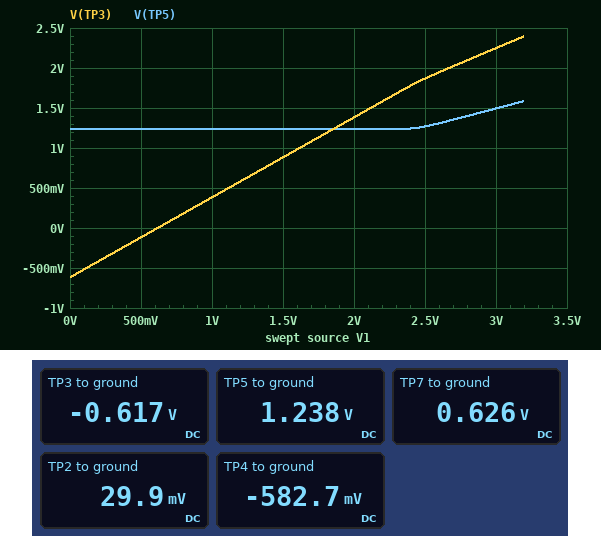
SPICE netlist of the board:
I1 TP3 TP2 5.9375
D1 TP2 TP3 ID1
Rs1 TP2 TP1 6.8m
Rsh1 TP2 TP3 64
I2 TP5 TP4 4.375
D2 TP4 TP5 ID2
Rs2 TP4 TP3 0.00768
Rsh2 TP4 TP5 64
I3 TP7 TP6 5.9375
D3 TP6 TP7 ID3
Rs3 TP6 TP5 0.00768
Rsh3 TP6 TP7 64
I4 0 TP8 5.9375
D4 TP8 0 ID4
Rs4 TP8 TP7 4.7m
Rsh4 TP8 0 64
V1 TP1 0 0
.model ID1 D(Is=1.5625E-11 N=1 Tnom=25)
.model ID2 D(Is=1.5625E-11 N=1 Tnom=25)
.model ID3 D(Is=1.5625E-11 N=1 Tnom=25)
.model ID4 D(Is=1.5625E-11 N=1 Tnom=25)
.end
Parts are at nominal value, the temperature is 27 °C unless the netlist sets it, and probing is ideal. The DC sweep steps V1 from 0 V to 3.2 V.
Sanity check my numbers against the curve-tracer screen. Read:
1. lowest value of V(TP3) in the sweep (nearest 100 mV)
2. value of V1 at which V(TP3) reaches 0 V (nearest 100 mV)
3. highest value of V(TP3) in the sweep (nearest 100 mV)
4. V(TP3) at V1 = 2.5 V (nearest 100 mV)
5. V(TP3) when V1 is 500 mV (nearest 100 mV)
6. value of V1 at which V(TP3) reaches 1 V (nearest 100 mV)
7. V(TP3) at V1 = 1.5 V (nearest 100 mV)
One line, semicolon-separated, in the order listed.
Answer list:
-600 mV; 600 mV; 2.4 V; 1.9 V; -100 mV; 1.6 V; 900 mV
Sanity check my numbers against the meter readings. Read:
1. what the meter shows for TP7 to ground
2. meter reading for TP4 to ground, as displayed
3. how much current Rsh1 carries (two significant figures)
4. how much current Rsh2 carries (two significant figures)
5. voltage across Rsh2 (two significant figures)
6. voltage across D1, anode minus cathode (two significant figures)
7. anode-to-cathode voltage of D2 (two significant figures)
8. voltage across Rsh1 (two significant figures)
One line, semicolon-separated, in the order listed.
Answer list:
0.626 V; -582.7 mV; 10 mA; 28 mA; 1.8 V; 650 mV; -1.8 V; 650 mV
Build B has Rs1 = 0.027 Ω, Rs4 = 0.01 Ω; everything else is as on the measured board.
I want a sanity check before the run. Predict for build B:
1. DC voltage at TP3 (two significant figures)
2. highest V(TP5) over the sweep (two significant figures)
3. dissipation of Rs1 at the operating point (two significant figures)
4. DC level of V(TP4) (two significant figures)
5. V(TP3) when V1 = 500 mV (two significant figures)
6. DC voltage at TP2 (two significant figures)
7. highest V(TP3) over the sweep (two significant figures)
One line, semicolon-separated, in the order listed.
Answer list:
-530 mV; 1.5 V; 520 mW; -490 mV; -28 mV; 120 mV; 2.3 V
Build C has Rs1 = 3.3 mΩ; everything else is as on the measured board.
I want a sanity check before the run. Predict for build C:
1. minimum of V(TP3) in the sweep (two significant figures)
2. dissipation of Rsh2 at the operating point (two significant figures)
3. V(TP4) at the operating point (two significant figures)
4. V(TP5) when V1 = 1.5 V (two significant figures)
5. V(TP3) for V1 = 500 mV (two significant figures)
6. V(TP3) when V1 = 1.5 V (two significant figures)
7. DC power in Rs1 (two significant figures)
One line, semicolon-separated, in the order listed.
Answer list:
-630 mV; 53 mW; -600 mV; 1.2 V; -130 mV; 870 mV; 64 mW
